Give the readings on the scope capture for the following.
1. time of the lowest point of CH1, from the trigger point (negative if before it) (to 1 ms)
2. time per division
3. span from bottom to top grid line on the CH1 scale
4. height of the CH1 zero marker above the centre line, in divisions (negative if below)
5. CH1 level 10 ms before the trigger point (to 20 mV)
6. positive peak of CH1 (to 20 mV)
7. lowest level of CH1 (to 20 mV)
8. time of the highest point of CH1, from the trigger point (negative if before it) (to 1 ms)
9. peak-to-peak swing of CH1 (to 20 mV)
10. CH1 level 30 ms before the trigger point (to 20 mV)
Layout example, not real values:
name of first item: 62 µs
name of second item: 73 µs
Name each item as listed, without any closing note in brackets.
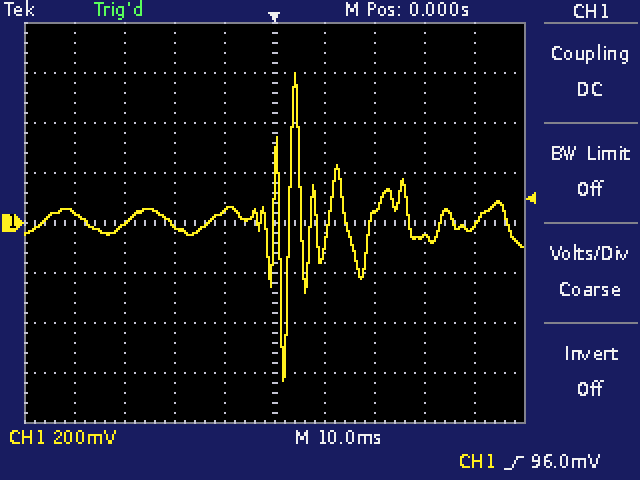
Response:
time of the lowest point of CH1, from the trigger point (negative if before it): +2 ms
time per division: 10 ms
span from bottom to top grid line on the CH1 scale: 1.6 V
height of the CH1 zero marker above the centre line, in divisions: 0.0 div
CH1 level 10 ms before the trigger point: 40 mV
positive peak of CH1: 600 mV
lowest level of CH1: -640 mV
time of the highest point of CH1, from the trigger point (negative if before it): +4 ms
peak-to-peak swing of CH1: 1.24 V
CH1 level 30 ms before the trigger point: 0 mV
